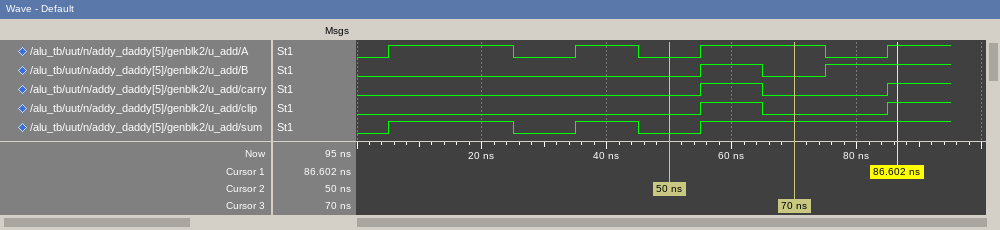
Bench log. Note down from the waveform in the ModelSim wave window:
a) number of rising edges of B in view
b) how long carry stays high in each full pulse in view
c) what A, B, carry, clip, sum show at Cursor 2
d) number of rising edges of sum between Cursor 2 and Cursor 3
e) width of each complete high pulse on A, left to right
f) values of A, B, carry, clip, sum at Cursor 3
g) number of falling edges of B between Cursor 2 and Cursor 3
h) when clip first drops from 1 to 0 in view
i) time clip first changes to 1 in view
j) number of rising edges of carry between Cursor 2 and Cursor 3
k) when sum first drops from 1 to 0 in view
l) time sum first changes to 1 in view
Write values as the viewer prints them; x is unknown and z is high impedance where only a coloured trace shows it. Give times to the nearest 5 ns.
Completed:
2
10 ns
A=0, B=0, carry=0, clip=0, sum=0
1
20 ns, 10 ns, 20 ns
A=1, B=0, carry=0, clip=0, sum=1
1
65 ns
55 ns
1
25 ns
5 ns
